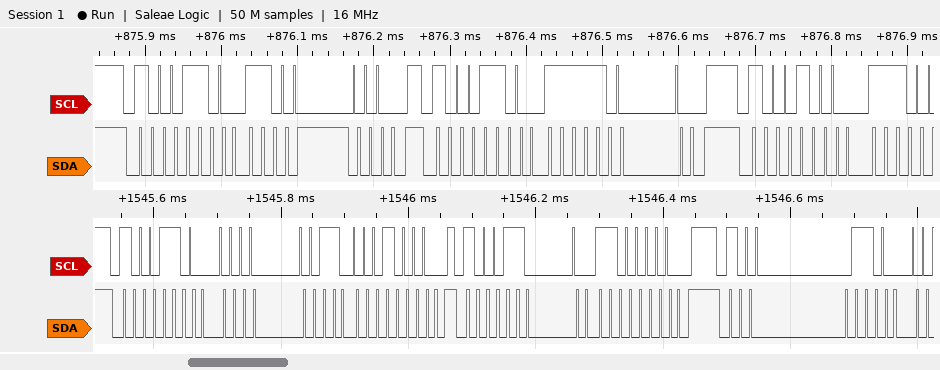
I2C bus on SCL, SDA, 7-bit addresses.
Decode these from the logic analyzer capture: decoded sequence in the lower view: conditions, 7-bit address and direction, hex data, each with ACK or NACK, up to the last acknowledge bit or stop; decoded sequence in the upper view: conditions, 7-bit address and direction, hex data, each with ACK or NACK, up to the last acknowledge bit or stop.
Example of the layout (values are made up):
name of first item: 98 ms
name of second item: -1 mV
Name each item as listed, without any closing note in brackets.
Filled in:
decoded sequence in the lower view: conditions, 7-bit address and direction, hex data, each with ACK or NACK, up to the last acknowledge bit or stop: start, address 46 write ACK, 03 ACK, 10 ACK, stop, start, address 46 write ACK, C0 ACK, stop, start, address 46 write ACK
decoded sequence in the upper view: conditions, 7-bit address and direction, hex data, each with ACK or NACK, up to the last acknowledge bit or stop: start, address 46 write ACK, C0 ACK, stop, start, address 46 write ACK, F8 ACK, stop, start, address 44 write ACK
